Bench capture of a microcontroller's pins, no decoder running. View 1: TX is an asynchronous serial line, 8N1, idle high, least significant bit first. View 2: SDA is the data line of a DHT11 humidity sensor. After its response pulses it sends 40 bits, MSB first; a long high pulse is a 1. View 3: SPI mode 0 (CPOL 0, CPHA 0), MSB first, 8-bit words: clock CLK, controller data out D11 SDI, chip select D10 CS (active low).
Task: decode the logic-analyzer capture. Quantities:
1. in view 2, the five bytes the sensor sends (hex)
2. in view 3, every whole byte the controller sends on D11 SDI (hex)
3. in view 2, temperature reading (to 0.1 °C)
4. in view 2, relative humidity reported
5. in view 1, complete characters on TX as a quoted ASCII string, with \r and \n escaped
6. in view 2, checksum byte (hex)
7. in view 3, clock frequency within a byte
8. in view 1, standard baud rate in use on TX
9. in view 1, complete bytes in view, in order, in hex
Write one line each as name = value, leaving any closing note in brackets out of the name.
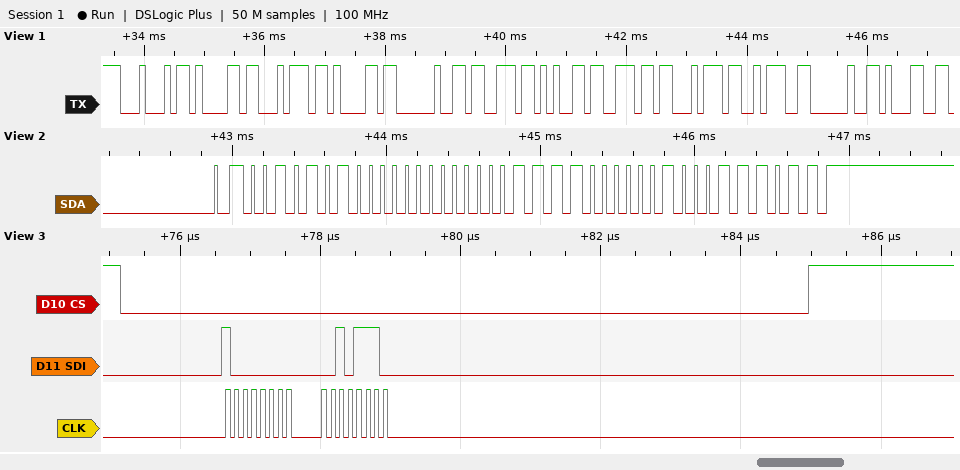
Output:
in view 2, the five bytes the sensor sends = 2A 00 0F 02 3B
in view 3, every whole byte the controller sends on D11 SDI = 80 2E
in view 2, temperature reading = 15.2 °C
in view 2, relative humidity reported = 42 %
in view 1, complete characters on TX as a quoted ASCII string, with \r and \n escaped = "Data sent: 1"
in view 2, checksum byte = 0x3B
in view 3, clock frequency within a byte = 8 MHz
in view 1, standard baud rate in use on TX = 9600 baud
in view 1, complete bytes in view, in order, in hex = 44 61 74 61 20 73 65 6E 74 3A 20 31
